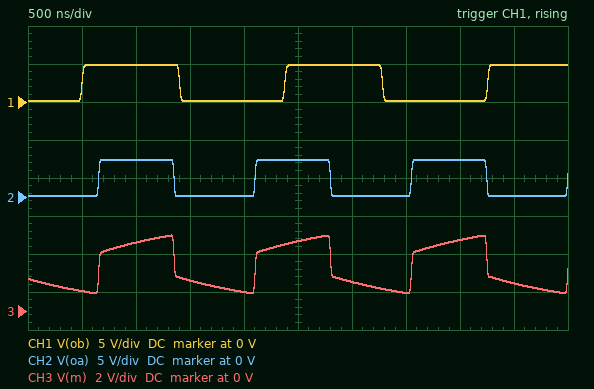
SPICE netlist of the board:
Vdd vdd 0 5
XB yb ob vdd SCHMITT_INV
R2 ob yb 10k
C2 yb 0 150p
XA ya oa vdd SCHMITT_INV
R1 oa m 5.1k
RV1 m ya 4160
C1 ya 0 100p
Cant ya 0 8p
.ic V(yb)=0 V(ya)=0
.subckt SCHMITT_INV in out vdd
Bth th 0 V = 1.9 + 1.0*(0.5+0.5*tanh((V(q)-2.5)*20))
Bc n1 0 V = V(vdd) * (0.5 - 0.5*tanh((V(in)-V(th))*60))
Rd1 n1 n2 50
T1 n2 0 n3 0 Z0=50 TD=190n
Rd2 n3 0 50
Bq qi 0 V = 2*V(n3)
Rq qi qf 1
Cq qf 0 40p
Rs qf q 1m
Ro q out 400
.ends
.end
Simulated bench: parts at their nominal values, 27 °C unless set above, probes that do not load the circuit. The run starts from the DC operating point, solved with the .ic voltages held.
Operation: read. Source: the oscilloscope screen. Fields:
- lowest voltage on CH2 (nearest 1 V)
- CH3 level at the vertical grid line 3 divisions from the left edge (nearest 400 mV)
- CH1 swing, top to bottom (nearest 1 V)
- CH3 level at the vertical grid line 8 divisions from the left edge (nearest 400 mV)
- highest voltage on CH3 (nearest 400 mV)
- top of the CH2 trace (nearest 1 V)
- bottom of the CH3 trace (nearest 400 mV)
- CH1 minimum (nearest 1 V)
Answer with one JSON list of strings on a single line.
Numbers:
["0 V", "1.6 V", "5 V", "3.6 V", "4.0 V", "5 V", "800 mV", "0 V"]
